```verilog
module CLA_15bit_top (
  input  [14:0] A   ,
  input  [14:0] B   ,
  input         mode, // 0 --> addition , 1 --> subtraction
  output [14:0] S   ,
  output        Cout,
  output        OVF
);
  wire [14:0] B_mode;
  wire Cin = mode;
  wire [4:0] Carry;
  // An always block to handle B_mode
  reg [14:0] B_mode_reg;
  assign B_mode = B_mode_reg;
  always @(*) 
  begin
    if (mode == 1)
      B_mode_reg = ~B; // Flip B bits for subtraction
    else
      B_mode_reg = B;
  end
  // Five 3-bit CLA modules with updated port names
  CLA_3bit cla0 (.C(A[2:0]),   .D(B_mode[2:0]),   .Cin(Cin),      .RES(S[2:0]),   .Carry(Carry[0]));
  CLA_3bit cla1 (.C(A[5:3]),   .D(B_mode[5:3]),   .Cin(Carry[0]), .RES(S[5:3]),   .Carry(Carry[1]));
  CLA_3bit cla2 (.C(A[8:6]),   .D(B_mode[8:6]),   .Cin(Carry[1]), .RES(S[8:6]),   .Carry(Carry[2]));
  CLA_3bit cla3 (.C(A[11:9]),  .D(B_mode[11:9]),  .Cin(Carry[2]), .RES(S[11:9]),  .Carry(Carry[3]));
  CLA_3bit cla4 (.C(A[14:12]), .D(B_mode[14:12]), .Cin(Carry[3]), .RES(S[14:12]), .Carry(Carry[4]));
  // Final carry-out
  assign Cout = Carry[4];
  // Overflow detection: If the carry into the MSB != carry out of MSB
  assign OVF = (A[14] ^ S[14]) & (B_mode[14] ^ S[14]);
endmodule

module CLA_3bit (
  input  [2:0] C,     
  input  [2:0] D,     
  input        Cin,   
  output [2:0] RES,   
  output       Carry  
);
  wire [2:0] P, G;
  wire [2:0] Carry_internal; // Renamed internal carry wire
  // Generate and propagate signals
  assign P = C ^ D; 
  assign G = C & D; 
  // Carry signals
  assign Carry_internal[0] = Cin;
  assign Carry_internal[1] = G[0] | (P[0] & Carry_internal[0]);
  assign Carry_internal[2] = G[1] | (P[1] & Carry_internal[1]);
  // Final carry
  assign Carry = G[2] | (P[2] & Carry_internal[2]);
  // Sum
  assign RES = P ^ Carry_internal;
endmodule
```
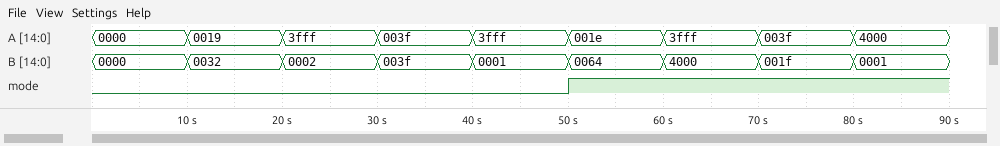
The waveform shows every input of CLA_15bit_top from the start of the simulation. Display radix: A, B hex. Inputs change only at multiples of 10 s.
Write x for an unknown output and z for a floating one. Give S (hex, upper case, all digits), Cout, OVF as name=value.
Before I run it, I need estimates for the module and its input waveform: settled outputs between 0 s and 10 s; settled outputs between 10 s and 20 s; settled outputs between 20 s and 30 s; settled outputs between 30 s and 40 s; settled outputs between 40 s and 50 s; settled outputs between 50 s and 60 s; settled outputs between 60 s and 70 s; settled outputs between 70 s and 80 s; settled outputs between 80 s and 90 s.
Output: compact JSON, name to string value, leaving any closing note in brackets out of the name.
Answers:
{"settled outputs between 0 s and 10 s": "S=0000, Cout=0, OVF=0", "settled outputs between 10 s and 20 s": "S=004B, Cout=0, OVF=0", "settled outputs between 20 s and 30 s": "S=4001, Cout=0, OVF=1", "settled outputs between 30 s and 40 s": "S=007E, Cout=0, OVF=0", "settled outputs between 40 s and 50 s": "S=4000, Cout=0, OVF=1", "settled outputs between 50 s and 60 s": "S=7FBA, Cout=0, OVF=0", "settled outputs between 60 s and 70 s": "S=7FFF, Cout=0, OVF=1", "settled outputs between 70 s and 80 s": "S=0020, Cout=1, OVF=0", "settled outputs between 80 s and 90 s": "S=3FFF, Cout=1, OVF=1"}
